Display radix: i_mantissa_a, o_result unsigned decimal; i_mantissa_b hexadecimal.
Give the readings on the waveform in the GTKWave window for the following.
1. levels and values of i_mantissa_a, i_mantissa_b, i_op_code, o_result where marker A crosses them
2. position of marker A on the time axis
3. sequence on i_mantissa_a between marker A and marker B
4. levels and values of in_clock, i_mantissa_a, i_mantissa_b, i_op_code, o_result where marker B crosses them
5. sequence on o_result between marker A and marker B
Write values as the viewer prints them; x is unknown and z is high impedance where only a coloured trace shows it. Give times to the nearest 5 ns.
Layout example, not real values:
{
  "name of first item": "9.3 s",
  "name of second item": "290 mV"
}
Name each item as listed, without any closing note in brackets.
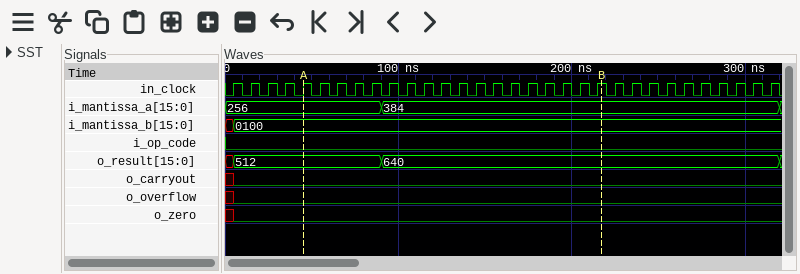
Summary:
{
  "levels and values of i_mantissa_a, i_mantissa_b, i_op_code, o_result where marker A crosses them": "i_mantissa_a=256, i_mantissa_b=0100, i_op_code=0, o_result=512",
  "position of marker A on the time axis": "45 ns",
  "sequence on i_mantissa_a between marker A and marker B": "256, 384",
  "levels and values of in_clock, i_mantissa_a, i_mantissa_b, i_op_code, o_result where marker B crosses them": "in_clock=1, i_mantissa_a=384, i_mantissa_b=0100, i_op_code=0, o_result=640",
  "sequence on o_result between marker A and marker B": "512, 640"
}
